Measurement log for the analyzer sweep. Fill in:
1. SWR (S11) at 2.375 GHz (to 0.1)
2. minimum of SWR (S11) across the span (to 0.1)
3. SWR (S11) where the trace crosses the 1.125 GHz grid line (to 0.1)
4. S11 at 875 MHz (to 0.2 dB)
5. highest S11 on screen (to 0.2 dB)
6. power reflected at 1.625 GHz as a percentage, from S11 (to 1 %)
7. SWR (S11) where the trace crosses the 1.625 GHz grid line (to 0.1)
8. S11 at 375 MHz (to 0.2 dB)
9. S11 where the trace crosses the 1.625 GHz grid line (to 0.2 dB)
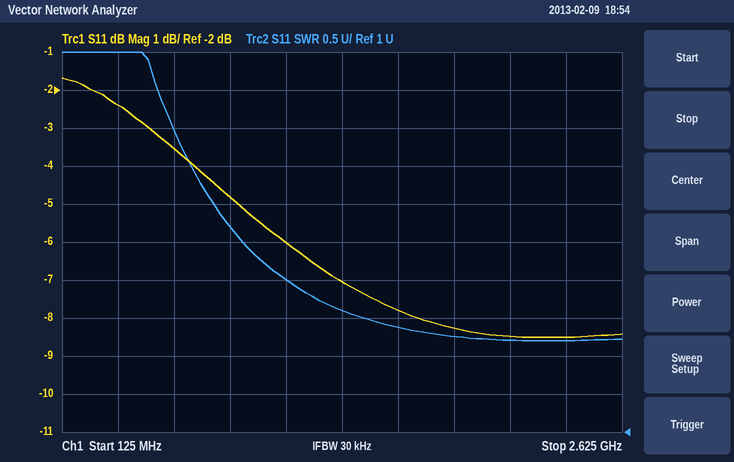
2.2
2.2
3.0
-4.8 dB
-1.6 dB
17 %
2.4
-2.4 dB
-7.8 dB
